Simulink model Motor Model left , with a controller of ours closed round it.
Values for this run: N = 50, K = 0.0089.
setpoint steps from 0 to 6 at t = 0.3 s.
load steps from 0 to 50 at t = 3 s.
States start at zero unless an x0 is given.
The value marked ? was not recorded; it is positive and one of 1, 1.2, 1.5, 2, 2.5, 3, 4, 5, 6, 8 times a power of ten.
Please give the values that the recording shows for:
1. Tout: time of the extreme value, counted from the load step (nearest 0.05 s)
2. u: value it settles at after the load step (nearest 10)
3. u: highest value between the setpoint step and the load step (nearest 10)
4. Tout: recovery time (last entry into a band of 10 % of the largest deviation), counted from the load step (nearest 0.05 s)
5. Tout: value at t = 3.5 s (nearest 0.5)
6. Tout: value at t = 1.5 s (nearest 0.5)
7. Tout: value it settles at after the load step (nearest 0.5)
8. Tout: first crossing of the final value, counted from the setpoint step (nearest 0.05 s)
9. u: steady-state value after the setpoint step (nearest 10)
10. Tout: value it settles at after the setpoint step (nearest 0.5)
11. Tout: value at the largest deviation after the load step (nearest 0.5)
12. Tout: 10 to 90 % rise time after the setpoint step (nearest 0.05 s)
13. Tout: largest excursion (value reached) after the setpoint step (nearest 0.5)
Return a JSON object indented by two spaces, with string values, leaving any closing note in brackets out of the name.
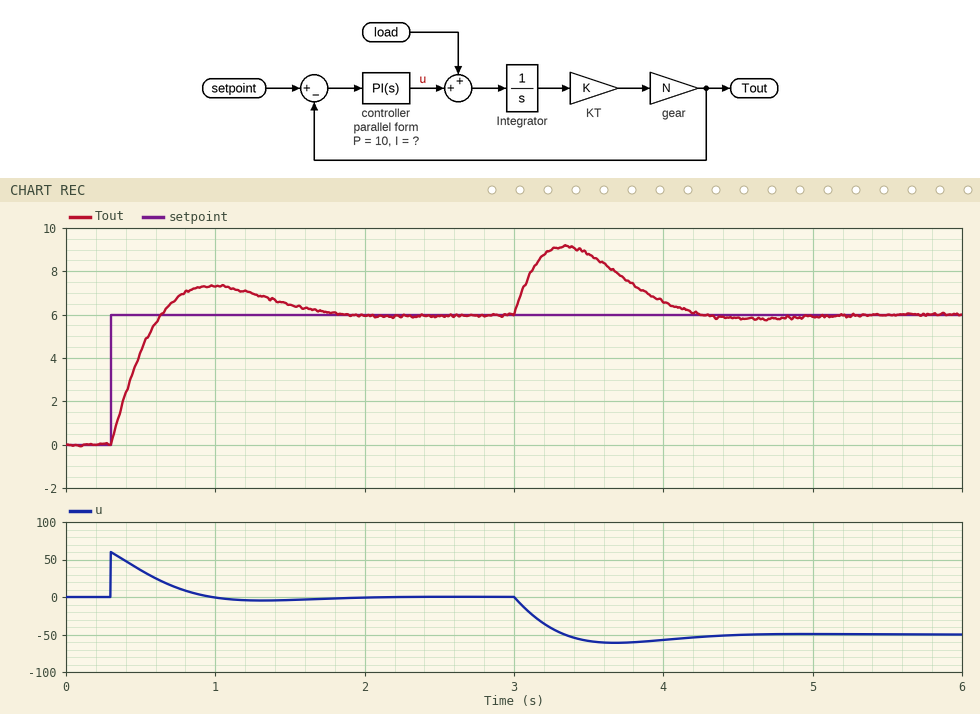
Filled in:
{
  "Tout: time of the extreme value, counted from the load step": "0.35 s",
  "u: value it settles at after the load step": "-50",
  "u: highest value between the setpoint step and the load step": "60",
  "Tout: recovery time (last entry into a band of 10 % of the largest deviation), counted from the load step": "1.10 s",
  "Tout: value at t = 3.5 s": "9.0",
  "Tout: value at t = 1.5 s": "6.5",
  "Tout: value it settles at after the load step": "6.0",
  "Tout: first crossing of the final value, counted from the setpoint step": "0.35 s",
  "u: steady-state value after the setpoint step": "0",
  "Tout: value it settles at after the setpoint step": "6.0",
  "Tout: value at the largest deviation after the load step": "9.0",
  "Tout: 10 to 90 % rise time after the setpoint step": "0.25 s",
  "Tout: largest excursion (value reached) after the setpoint step": "7.5"
}
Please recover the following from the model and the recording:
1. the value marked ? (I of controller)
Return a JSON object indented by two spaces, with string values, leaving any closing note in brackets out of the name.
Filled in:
{
  "the value marked ?": "25"
}
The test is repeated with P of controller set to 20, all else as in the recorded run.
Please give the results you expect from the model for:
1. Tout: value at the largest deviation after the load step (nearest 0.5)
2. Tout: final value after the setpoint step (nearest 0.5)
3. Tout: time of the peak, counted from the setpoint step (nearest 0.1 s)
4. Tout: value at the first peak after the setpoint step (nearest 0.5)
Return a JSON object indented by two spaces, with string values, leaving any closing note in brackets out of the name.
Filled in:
{
  "Tout: value at the largest deviation after the load step": "8.0",
  "Tout: final value after the setpoint step": "6.0",
  "Tout: time of the peak, counted from the setpoint step": "0.5 s",
  "Tout: value at the first peak after the setpoint step": "6.5"
}
